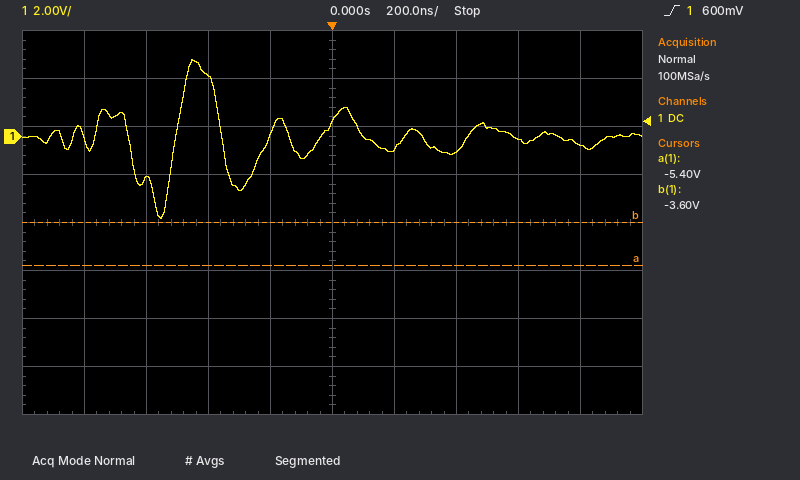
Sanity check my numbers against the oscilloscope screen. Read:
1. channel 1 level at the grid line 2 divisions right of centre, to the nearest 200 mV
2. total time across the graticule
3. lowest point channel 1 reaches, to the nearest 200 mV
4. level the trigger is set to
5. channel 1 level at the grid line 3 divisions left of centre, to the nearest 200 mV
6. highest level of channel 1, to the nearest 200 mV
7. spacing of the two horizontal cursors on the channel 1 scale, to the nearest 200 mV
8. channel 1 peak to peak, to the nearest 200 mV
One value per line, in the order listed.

-600 mV
2 µs
-3.4 V
600 mV
-1.8 V
3.2 V
1.8 V
6.6 V
